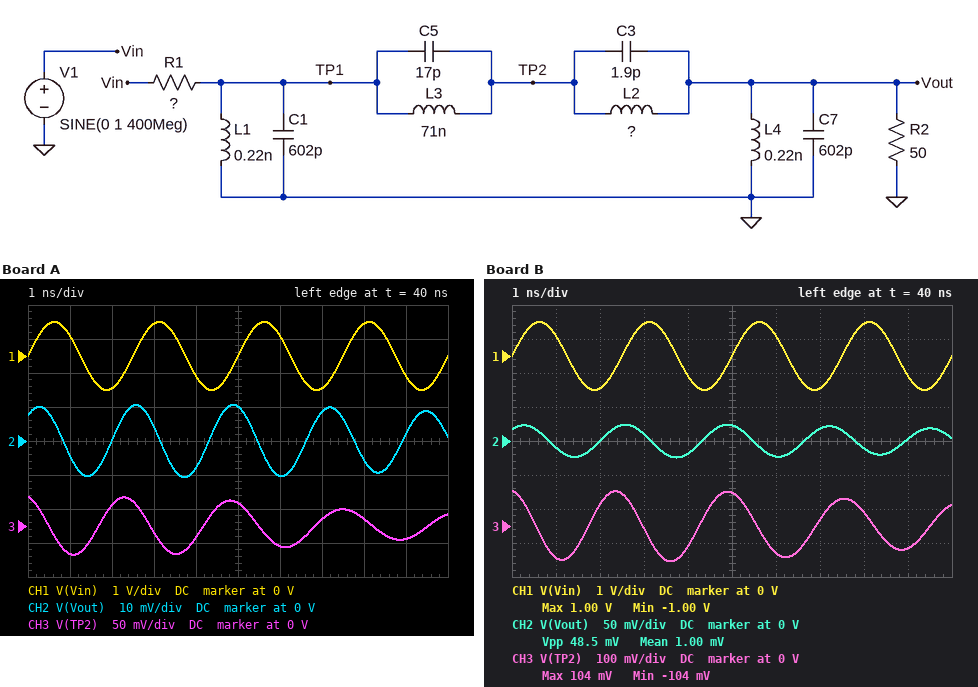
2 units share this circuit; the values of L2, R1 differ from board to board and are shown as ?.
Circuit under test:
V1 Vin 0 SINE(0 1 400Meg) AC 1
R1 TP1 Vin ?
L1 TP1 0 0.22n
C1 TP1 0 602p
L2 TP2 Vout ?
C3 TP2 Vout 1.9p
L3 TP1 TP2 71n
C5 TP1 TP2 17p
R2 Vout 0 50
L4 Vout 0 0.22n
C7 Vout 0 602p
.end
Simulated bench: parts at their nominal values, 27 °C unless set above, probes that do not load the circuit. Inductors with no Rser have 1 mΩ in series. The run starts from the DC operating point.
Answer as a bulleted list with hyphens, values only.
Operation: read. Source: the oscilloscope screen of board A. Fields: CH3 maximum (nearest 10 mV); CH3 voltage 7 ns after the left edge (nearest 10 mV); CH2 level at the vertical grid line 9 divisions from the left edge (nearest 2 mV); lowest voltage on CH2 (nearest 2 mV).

- 40 mV
- 10 mV
- 2 mV
- -10 mV
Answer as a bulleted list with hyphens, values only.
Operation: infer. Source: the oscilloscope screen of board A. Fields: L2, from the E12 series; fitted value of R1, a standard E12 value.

- 18 nH
- 150 Ω
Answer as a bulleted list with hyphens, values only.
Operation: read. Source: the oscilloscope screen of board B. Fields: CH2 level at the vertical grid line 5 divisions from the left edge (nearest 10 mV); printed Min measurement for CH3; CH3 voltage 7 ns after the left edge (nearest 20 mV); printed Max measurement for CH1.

- 20 mV
- -104 mV
- 20 mV
- 1.00 V
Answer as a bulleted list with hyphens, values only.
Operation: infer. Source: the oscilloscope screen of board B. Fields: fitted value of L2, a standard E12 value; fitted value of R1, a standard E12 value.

- 18 nH
- 56 Ω
